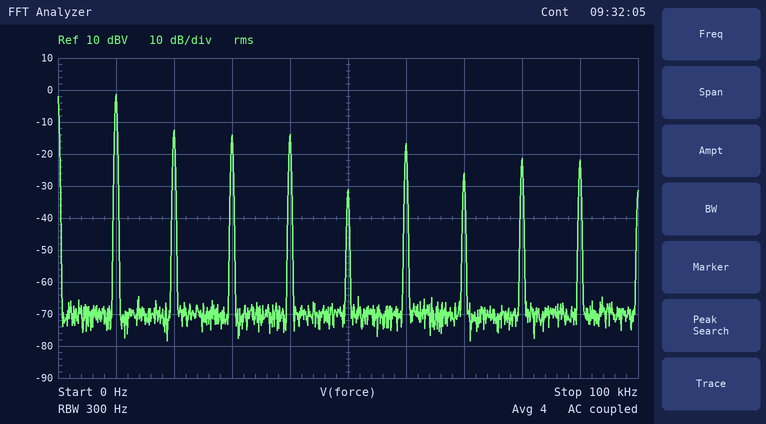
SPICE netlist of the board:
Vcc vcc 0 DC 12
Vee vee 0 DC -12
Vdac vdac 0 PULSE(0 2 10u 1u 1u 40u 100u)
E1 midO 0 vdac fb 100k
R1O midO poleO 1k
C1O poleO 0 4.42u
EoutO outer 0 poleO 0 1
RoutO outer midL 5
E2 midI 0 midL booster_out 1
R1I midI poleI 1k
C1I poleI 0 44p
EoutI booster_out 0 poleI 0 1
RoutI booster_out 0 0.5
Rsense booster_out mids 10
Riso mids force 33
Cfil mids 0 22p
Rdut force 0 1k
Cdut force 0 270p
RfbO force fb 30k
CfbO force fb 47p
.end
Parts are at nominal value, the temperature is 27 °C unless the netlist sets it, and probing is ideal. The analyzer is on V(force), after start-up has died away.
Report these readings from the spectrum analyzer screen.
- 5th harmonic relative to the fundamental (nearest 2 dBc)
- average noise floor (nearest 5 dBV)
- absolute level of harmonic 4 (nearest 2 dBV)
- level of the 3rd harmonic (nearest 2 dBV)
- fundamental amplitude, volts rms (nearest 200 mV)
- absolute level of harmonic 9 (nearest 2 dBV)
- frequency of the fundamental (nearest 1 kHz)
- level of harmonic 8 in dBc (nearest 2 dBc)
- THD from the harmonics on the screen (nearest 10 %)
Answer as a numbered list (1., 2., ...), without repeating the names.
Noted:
1. -30 dBc
2. -70 dBV
3. -14 dBV
4. -14 dBV
5. 800 mV
6. -22 dBV
7. 10 kHz
8. -20 dBc
9. 50 %
